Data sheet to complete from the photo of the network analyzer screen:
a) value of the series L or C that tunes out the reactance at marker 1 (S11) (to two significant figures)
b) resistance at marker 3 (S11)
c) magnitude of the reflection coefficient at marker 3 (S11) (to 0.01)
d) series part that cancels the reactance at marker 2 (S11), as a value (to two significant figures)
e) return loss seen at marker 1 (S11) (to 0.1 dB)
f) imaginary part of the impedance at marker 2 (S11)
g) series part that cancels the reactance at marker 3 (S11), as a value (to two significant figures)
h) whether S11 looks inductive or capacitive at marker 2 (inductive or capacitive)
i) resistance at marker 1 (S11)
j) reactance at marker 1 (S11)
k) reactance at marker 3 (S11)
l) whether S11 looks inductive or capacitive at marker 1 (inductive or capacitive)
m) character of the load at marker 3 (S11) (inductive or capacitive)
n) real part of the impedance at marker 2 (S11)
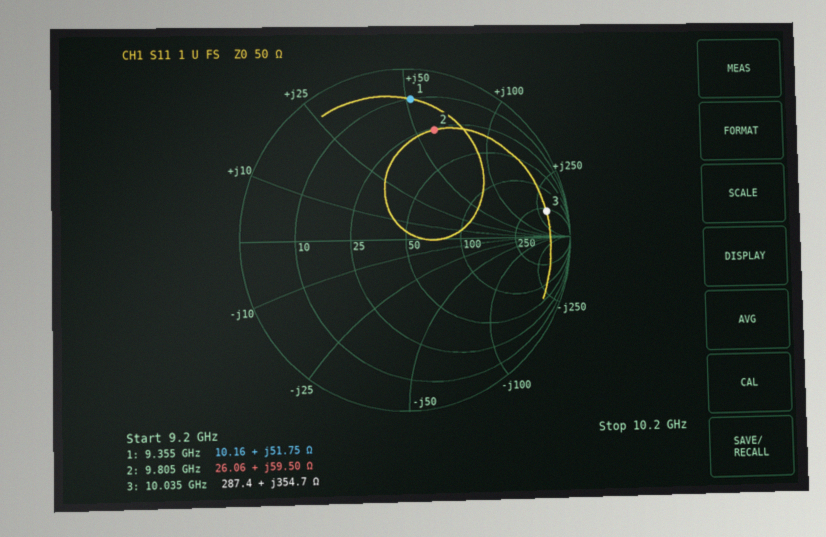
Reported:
330 fF
287.4 Ω
0.87
270 fF
1.7 dB
+59.50 Ω
45 fF
inductive
10.16 Ω
+51.75 Ω
+354.7 Ω
inductive
inductive
26.06 Ω
